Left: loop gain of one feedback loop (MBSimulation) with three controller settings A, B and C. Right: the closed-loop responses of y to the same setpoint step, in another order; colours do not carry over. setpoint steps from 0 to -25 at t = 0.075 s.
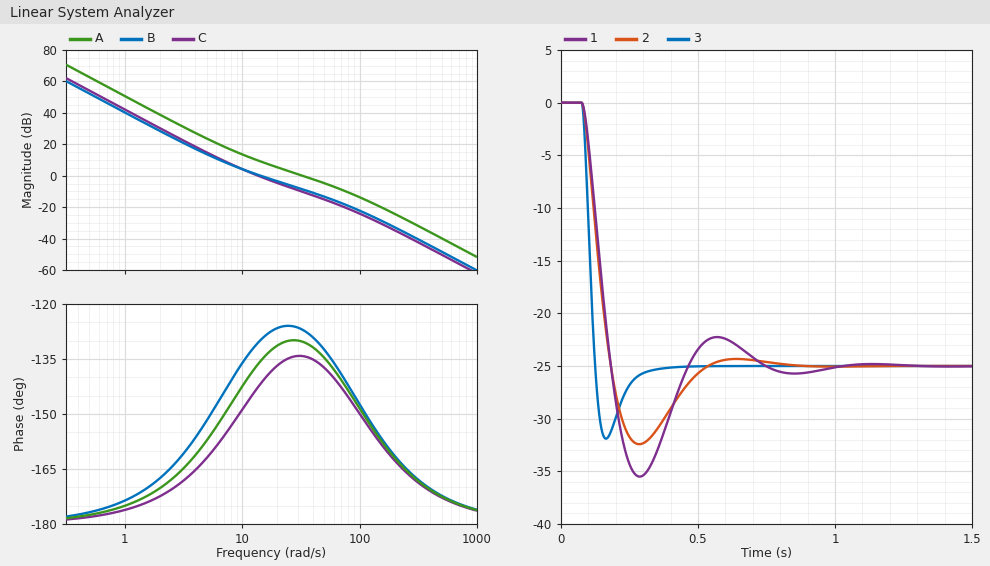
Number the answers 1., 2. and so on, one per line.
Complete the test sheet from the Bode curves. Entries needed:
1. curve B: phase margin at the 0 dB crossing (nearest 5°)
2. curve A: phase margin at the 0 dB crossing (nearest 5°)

1. 50°
2. 50°
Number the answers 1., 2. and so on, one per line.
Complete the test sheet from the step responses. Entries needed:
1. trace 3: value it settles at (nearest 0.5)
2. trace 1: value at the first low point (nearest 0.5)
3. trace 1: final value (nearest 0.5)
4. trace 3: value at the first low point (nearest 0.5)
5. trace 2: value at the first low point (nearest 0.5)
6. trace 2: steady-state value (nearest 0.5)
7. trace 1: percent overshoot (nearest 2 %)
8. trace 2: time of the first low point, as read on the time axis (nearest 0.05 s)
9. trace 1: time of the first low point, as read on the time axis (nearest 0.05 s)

1. -25.0
2. -35.5
3. -25.0
4. -32.0
5. -32.5
6. -25.0
7. 42 %
8. 0.30 s
9. 0.30 s
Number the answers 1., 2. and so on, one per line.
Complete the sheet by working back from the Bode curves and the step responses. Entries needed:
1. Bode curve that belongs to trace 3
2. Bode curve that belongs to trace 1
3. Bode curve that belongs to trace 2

1. A
2. C
3. B
